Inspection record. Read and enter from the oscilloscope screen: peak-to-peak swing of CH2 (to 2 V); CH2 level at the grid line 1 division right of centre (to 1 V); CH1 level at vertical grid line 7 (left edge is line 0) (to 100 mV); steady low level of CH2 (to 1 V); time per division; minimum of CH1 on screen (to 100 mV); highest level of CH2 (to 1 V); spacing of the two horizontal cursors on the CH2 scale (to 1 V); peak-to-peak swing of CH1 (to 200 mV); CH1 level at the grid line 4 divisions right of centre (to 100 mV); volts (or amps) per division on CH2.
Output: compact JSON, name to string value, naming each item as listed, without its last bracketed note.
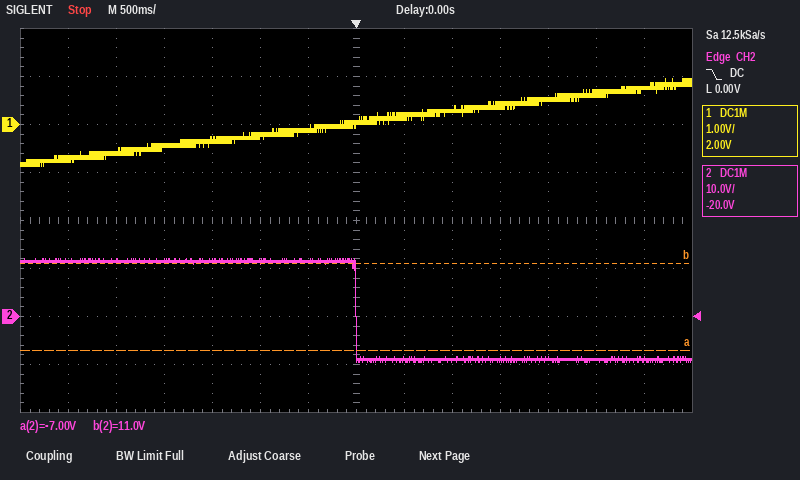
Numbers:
{"peak-to-peak swing of CH2": "22 V", "CH2 level at the grid line 1 division right of centre": "-9 V", "CH1 level at vertical grid line 7 (left edge is line 0)": "0.0 V", "steady low level of CH2": "-9 V", "time per division": "500 ms", "minimum of CH1 on screen": "-900 mV", "highest level of CH2": "12 V", "spacing of the two horizontal cursors on the CH2 scale": "18 V", "peak-to-peak swing of CH1": "1.8 V", "CH1 level at the grid line 4 divisions right of centre": "500 mV", "volts (or amps) per division on CH2": "10 V"}
